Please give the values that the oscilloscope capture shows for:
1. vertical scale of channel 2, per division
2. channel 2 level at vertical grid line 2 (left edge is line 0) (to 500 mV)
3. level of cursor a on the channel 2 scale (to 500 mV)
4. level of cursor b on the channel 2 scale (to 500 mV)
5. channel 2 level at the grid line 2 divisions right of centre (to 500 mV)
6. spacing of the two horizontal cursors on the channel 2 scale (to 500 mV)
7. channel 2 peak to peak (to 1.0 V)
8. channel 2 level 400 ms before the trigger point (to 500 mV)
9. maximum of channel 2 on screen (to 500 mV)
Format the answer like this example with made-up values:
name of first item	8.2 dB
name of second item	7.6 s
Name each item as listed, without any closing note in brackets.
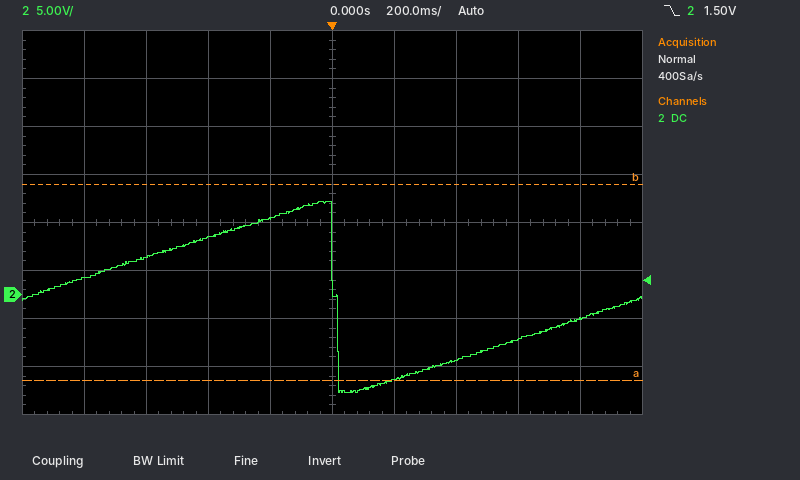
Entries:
vertical scale of channel 2, per division	5 V
channel 2 level at vertical grid line 2 (left edge is line 0)	4.0 V
level of cursor a on the channel 2 scale	-9.0 V
level of cursor b on the channel 2 scale	11.5 V
channel 2 level at the grid line 2 divisions right of centre	-7.0 V
spacing of the two horizontal cursors on the channel 2 scale	20.5 V
channel 2 peak to peak	20.0 V
channel 2 level 400 ms before the trigger point	6.0 V
maximum of channel 2 on screen	9.5 V
